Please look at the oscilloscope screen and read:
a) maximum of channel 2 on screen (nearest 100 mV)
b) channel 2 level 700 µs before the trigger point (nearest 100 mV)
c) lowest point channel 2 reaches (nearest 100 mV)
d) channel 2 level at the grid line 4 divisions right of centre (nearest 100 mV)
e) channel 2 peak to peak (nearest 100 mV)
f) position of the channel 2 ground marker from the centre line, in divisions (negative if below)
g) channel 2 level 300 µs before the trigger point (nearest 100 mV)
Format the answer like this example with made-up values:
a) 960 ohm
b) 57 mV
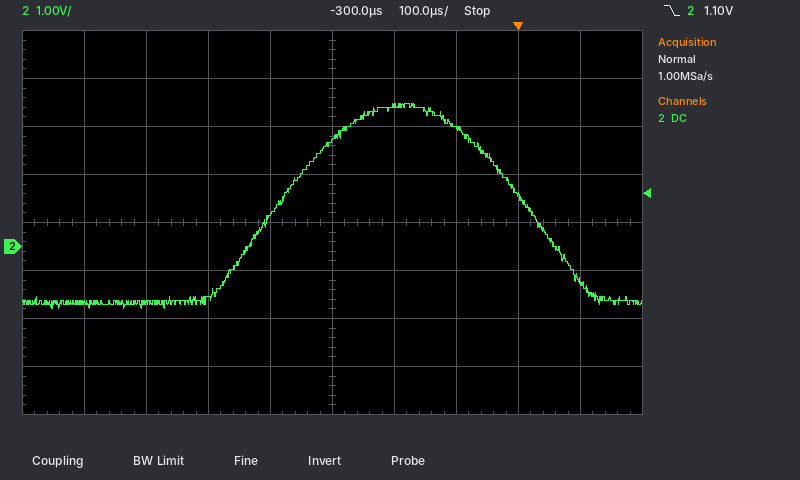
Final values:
a) 3.0 V
b) -1.2 V
c) -1.3 V
d) -700 mV
e) 4.3 V
f) -0.5 div
g) 2.2 V
